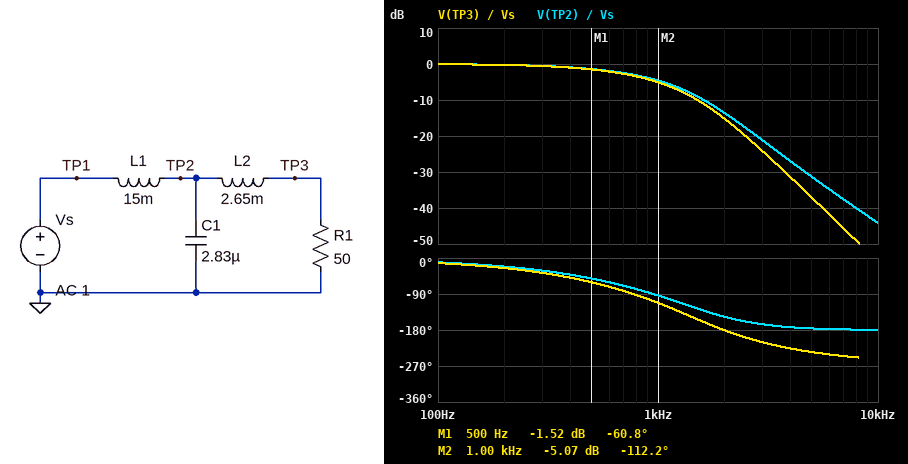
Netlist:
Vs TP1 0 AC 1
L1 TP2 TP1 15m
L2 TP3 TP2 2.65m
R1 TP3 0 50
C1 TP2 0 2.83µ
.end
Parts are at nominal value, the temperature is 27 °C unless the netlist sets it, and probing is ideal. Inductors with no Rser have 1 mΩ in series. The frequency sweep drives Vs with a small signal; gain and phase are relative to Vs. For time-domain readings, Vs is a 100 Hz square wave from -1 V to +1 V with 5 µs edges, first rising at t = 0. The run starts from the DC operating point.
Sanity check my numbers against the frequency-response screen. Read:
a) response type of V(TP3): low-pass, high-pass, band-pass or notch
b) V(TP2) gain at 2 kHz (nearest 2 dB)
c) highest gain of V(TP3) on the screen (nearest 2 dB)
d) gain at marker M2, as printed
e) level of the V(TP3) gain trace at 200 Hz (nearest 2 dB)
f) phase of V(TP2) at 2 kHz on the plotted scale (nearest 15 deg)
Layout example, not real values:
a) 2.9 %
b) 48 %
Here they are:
a) low-pass
b) -14 dB
c) 0 dB
d) -5.07 dB
e) 0 dB
f) -150 deg
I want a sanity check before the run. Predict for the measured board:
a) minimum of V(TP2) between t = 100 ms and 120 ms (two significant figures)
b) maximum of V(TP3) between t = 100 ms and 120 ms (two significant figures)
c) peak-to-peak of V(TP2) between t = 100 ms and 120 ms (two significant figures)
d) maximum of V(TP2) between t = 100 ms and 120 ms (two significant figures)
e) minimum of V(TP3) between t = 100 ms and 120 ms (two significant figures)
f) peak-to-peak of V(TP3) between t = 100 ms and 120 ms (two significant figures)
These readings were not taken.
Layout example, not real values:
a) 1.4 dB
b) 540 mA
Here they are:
a) -1.0 V
b) 1.0 V
c) 2.0 V
d) 1.0 V
e) -1.0 V
f) 2.0 V
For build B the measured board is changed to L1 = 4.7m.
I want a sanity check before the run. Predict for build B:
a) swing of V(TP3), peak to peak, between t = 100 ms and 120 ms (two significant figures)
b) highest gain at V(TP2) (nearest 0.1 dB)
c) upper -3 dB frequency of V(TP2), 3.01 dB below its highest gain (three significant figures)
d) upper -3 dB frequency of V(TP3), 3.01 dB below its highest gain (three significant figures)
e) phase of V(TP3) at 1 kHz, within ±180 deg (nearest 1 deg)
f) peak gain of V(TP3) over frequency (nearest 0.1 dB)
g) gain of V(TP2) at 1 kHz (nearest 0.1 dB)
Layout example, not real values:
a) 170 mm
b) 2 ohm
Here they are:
a) 2.8 V
b) 2.7 dB
c) 2.04 kHz
d) 1.97 kHz
e) -58 deg
f) 1.8 dB
g) 1.5 dB
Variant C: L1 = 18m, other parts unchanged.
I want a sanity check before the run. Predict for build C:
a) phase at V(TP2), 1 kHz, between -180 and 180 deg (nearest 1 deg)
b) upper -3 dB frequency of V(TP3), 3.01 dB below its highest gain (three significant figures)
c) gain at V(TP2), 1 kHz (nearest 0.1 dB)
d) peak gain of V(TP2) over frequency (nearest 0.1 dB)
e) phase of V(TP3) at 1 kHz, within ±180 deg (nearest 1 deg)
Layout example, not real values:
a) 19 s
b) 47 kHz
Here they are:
a) -99 deg
b) 582 Hz
c) -6.3 dB
d) 0 dB
e) -118 deg
